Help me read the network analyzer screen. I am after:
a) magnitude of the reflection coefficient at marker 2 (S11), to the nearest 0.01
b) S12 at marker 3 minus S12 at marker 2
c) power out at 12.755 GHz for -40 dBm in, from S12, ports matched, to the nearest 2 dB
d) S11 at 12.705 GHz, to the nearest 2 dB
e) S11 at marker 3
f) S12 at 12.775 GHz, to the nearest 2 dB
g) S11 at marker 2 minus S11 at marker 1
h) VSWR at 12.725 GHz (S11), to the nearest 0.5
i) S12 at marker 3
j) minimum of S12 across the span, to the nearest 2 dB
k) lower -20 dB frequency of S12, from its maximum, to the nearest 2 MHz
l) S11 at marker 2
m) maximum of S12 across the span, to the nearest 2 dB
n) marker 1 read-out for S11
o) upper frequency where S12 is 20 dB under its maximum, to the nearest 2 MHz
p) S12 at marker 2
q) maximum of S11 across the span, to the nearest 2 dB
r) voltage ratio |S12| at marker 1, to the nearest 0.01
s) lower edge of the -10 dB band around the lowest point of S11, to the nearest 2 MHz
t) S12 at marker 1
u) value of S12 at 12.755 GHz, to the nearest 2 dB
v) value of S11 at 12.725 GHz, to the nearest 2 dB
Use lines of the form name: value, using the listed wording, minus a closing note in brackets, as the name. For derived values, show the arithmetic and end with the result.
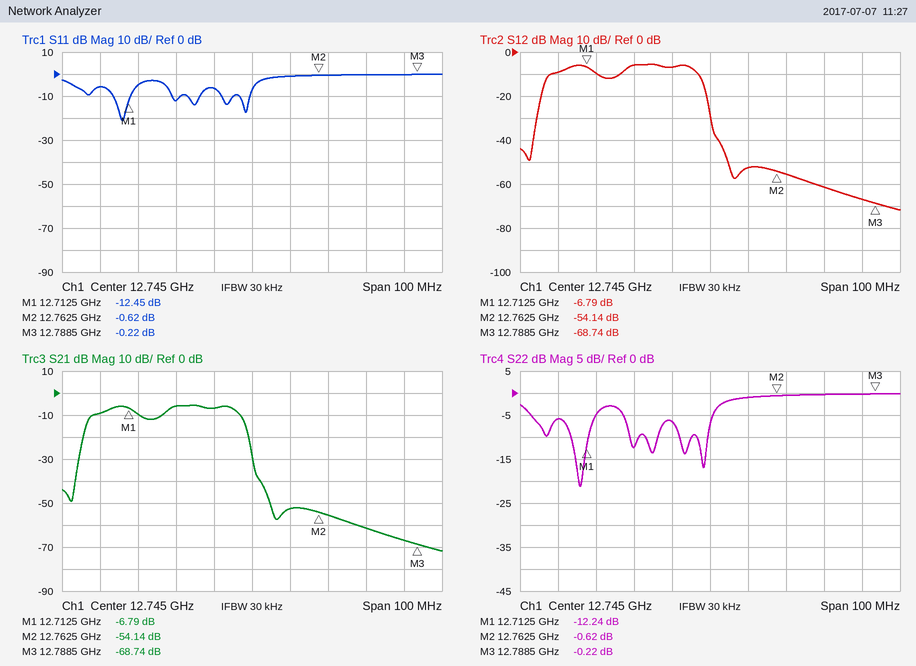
magnitude of the reflection coefficient at marker 2 (S11), to the nearest 0.01: 10^(-0.62/20) ≈ 0.93
S12 at marker 3 minus S12 at marker 2: -68.74 − (-54.14) = -14.60 dB
power out at 12.755 GHz for -40 dBm in, from S12, ports matched, to the nearest 2 dB: -40 dBm + (-52 dB) = -92 dBm
S11 at 12.705 GHz, to the nearest 2 dB: -6 dB
S11 at marker 3: -0.22 dB
S12 at 12.775 GHz, to the nearest 2 dB: -62 dB
S11 at marker 2 minus S11 at marker 1: -0.62 − (-12.45) = 11.83 dB
VSWR at 12.725 GHz (S11), to the nearest 0.5: |Γ| = 10^(-12/20) = 0.2512; VSWR = (1 + 0.2512)/(1 − 0.2512) ≈ 1.67, so 1.5 to the nearest 0.5
S12 at marker 3: -68.74 dB
minimum of S12 across the span, to the nearest 2 dB: -72 dB
lower -20 dB frequency of S12, from its maximum, to the nearest 2 MHz: 12.700 GHz
S11 at marker 2: -0.62 dB
maximum of S12 across the span, to the nearest 2 dB: -6 dB
marker 1 read-out for S11: -12.45 dB
upper frequency where S12 is 20 dB under its maximum, to the nearest 2 MHz: 12.744 GHz
S12 at marker 2: -54.14 dB
maximum of S11 across the span, to the nearest 2 dB: 0 dB
voltage ratio |S12| at marker 1, to the nearest 0.01: 10^(-6.79/20) ≈ 0.46
lower edge of the -10 dB band around the lowest point of S11, to the nearest 2 MHz: 12.708 GHz
S12 at marker 1: -6.79 dB
value of S12 at 12.755 GHz, to the nearest 2 dB: -52 dB
value of S11 at 12.725 GHz, to the nearest 2 dB: -12 dB
